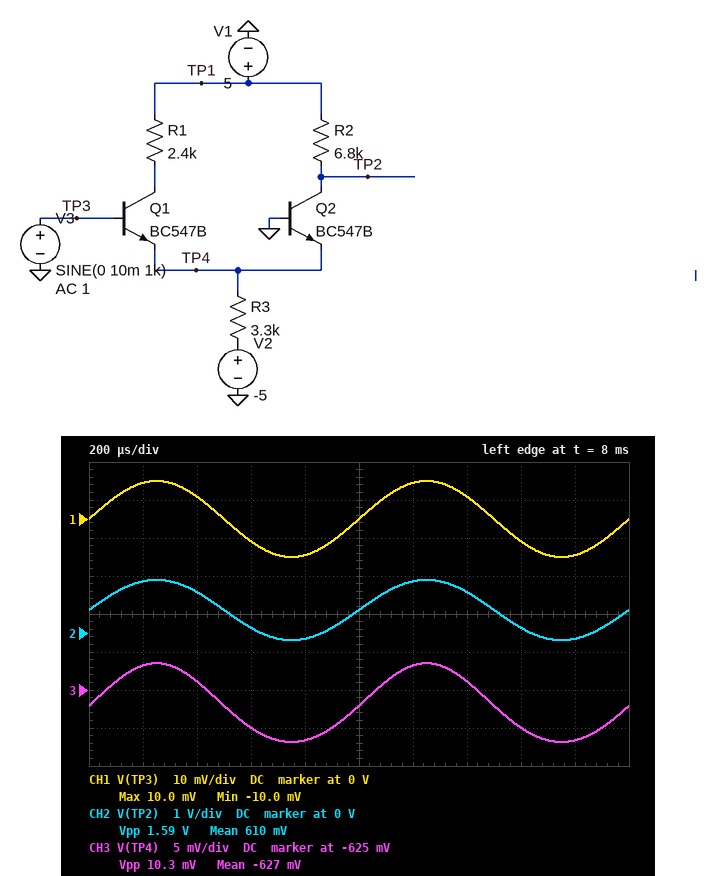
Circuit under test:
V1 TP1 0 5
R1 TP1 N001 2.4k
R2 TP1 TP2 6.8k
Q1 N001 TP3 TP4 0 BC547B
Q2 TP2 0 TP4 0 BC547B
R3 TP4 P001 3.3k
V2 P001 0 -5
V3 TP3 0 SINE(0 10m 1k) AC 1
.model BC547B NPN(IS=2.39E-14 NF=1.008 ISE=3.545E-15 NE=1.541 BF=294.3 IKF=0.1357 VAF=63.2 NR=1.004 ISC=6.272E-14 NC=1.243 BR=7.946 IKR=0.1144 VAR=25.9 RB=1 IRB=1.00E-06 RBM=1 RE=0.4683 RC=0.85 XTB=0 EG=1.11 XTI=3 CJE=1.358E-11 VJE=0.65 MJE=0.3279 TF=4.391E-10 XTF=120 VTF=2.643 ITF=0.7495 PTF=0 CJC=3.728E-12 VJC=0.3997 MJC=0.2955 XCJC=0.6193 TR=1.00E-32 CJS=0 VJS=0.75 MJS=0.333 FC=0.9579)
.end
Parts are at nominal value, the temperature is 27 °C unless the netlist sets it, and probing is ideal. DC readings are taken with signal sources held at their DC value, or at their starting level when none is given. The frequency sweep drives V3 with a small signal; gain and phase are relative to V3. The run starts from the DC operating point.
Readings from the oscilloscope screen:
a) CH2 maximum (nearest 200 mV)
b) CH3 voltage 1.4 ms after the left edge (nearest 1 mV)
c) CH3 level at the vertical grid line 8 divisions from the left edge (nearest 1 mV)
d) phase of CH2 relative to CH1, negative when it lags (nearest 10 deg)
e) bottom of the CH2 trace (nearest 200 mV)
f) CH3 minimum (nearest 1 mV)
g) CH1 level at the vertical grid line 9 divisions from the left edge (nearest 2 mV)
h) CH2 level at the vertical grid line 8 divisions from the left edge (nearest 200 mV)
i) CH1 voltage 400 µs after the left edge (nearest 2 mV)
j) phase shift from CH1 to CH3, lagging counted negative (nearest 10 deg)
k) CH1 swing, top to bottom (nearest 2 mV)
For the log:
1.4 V
-624 mV
-630 mV
0 deg
-200 mV
-632 mV
-10 mV
200 mV
6 mV
0 deg
20 mV
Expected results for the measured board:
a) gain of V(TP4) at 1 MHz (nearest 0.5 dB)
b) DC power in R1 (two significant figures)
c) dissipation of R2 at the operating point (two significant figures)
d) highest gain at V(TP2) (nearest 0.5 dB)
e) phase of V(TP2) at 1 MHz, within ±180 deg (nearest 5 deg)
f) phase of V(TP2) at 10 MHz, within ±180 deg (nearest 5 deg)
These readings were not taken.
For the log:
-5.5 dB
1.1 mW
2.8 mW
38.0 dB
-5 deg
-50 deg
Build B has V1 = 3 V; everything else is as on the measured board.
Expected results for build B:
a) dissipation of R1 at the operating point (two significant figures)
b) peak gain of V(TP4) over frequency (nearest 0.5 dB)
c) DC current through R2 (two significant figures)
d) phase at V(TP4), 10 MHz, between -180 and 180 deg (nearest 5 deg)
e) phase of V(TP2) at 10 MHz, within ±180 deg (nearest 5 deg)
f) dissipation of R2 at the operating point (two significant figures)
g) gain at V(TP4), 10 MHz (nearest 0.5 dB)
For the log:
1.4 mW
-1.5 dB
530 µA
-15 deg
-35 deg
1.9 mW
-2.5 dB
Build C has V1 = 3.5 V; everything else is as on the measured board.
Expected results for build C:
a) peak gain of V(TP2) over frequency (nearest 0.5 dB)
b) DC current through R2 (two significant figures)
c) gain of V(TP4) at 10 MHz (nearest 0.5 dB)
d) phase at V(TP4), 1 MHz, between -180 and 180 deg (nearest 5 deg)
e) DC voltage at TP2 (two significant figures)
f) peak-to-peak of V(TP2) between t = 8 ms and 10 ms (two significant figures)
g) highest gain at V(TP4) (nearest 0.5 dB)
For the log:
16.0 dB
600 µA
-4.0 dB
-5 deg
-570 mV
500 mV
-1.5 dB
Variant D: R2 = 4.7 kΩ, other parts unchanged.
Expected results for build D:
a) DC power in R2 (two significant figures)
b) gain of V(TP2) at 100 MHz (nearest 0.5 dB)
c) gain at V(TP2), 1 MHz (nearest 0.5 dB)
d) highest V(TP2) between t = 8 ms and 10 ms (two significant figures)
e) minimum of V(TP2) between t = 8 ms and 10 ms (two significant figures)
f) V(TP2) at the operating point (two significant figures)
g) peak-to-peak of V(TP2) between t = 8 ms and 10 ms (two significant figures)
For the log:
2.0 mW
18.5 dB
35.0 dB
2.5 V
1.4 V
1.9 V
1.1 V
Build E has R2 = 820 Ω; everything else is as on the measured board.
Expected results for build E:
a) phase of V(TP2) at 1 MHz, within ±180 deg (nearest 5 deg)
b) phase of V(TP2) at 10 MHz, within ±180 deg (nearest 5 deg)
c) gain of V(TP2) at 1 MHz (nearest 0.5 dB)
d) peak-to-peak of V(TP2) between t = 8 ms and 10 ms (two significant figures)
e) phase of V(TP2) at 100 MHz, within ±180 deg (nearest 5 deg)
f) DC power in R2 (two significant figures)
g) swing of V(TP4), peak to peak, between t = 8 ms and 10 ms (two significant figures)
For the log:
0 deg
-5 deg
20.0 dB
200 mV
-45 deg
360 µW
9.8 mV
